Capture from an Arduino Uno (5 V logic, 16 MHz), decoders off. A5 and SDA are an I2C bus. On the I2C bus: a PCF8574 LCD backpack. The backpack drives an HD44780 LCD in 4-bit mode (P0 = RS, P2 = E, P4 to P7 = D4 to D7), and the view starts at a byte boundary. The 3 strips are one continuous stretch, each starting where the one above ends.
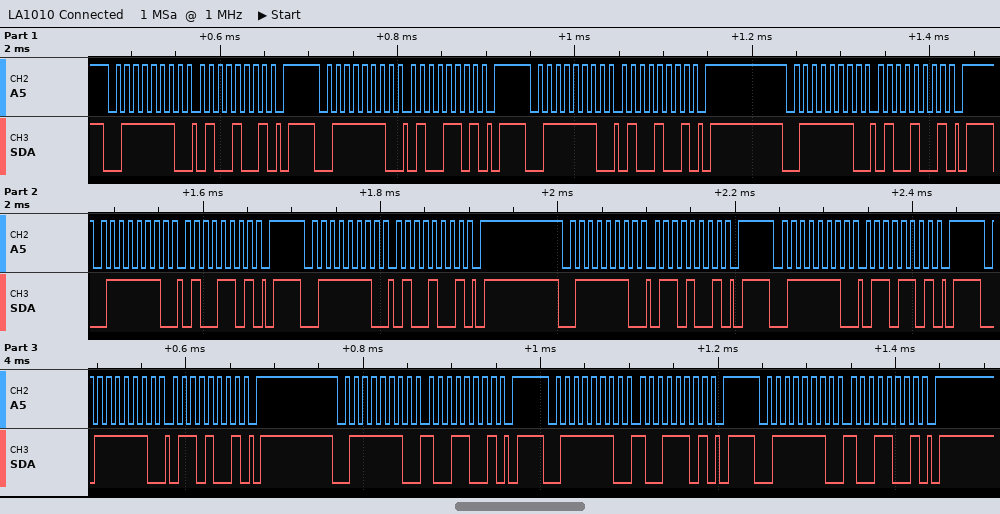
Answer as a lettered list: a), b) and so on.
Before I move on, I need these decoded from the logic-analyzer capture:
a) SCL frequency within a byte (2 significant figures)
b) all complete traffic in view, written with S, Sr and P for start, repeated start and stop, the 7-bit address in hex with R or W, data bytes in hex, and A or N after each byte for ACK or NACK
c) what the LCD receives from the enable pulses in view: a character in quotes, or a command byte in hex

a) 100 kHz
b) S 3FW A 49 A P S 3FW A 4D A P S 3FW A 49 A P S 3FW A 49 A P S 3FW A 4D A P S 3FW A 49 A P S 3FW A 69 A P S 3FW A 6D A P S 3FW A 69 A P S 3FW A 99 A P S 3FW A 9D A P S 3FW A 99 A P
c) 'D' 'i'
